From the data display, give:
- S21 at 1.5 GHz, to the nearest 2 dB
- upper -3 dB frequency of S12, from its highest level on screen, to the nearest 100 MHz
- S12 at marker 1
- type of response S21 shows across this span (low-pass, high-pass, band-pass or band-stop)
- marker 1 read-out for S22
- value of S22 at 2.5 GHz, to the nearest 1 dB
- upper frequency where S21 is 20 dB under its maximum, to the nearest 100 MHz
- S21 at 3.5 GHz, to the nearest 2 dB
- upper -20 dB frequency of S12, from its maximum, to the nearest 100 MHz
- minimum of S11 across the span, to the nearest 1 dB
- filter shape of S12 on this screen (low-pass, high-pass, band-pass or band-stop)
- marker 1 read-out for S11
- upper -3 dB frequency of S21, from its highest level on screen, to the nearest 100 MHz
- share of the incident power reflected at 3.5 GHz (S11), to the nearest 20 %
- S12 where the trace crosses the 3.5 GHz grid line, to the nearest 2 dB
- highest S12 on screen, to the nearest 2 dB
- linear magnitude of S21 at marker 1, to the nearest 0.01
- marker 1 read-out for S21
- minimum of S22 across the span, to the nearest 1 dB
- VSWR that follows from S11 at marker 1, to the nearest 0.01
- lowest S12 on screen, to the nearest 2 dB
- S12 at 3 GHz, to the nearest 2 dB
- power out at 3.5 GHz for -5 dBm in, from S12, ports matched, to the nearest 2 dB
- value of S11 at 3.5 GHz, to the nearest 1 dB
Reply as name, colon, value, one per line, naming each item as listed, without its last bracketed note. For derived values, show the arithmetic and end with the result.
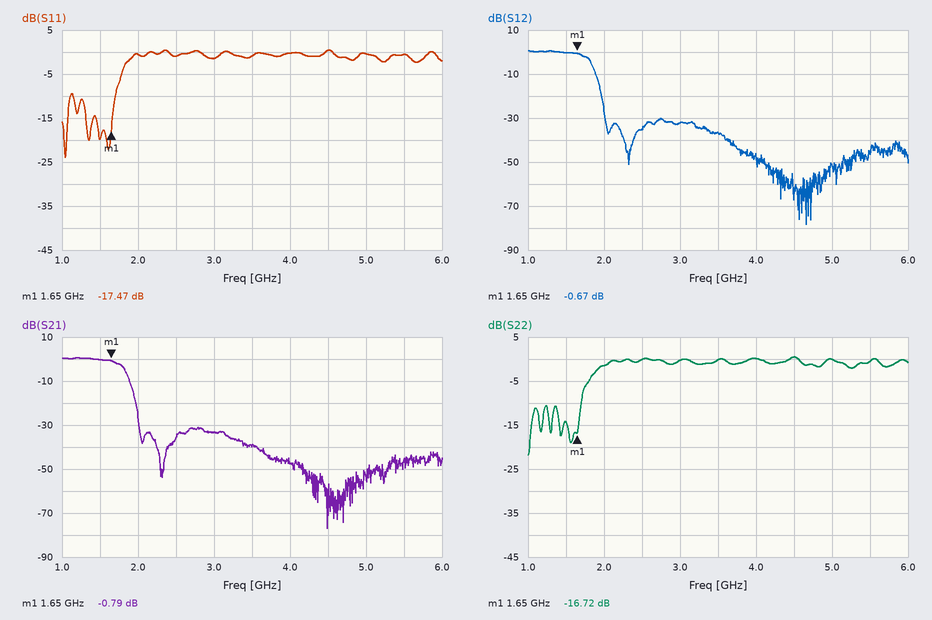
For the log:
S21 at 1.5 GHz, to the nearest 2 dB: 0 dB
upper -3 dB frequency of S12, from its highest level on screen, to the nearest 100 MHz: 1.8 GHz
S12 at marker 1: -0.67 dB
type of response S21 shows across this span: low-pass
marker 1 read-out for S22: -16.72 dB
value of S22 at 2.5 GHz, to the nearest 1 dB: 0 dB
upper frequency where S21 is 20 dB under its maximum, to the nearest 100 MHz: 2.0 GHz
S21 at 3.5 GHz, to the nearest 2 dB: -40 dB
upper -20 dB frequency of S12, from its maximum, to the nearest 100 MHz: 2.0 GHz
minimum of S11 across the span, to the nearest 1 dB: -24 dB
filter shape of S12 on this screen: low-pass
marker 1 read-out for S11: -17.47 dB
upper -3 dB frequency of S21, from its highest level on screen, to the nearest 100 MHz: 1.8 GHz
share of the incident power reflected at 3.5 GHz (S11), to the nearest 20 %: 10^(-1/10) ≈ 79.4 %, so 80 % to the nearest 20 %
S12 where the trace crosses the 3.5 GHz grid line, to the nearest 2 dB: -36 dB
highest S12 on screen, to the nearest 2 dB: 0 dB
linear magnitude of S21 at marker 1, to the nearest 0.01: 10^(-0.79/20) ≈ 0.91
marker 1 read-out for S21: -0.79 dB
minimum of S22 across the span, to the nearest 1 dB: -22 dB
VSWR that follows from S11 at marker 1, to the nearest 0.01: (1 + 0.1338)/(1 − 0.1338) ≈ 1.31
lowest S12 on screen, to the nearest 2 dB: -78 dB
S12 at 3 GHz, to the nearest 2 dB: -32 dB
power out at 3.5 GHz for -5 dBm in, from S12, ports matched, to the nearest 2 dB: -5 dBm + (-36 dB) = -42 dBm
value of S11 at 3.5 GHz, to the nearest 1 dB: -1 dB
